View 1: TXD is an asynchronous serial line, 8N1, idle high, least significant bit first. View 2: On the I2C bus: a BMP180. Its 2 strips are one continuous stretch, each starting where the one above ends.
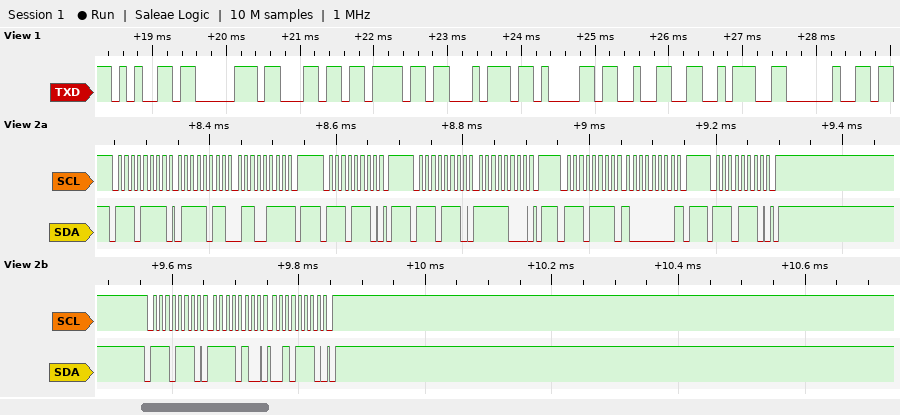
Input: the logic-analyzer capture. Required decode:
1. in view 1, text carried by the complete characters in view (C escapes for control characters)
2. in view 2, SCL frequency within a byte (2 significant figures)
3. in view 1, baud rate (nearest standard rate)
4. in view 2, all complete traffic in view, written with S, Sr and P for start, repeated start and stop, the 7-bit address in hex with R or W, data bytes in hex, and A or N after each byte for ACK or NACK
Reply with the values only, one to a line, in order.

"eplota2: "
100 kHz
9600 baud
S 77R A 7B A 67 N P S 77W A P S 77W A F8 A P S 77R A 80 N P S 77W A P S 77W A F4 A 2E A P
